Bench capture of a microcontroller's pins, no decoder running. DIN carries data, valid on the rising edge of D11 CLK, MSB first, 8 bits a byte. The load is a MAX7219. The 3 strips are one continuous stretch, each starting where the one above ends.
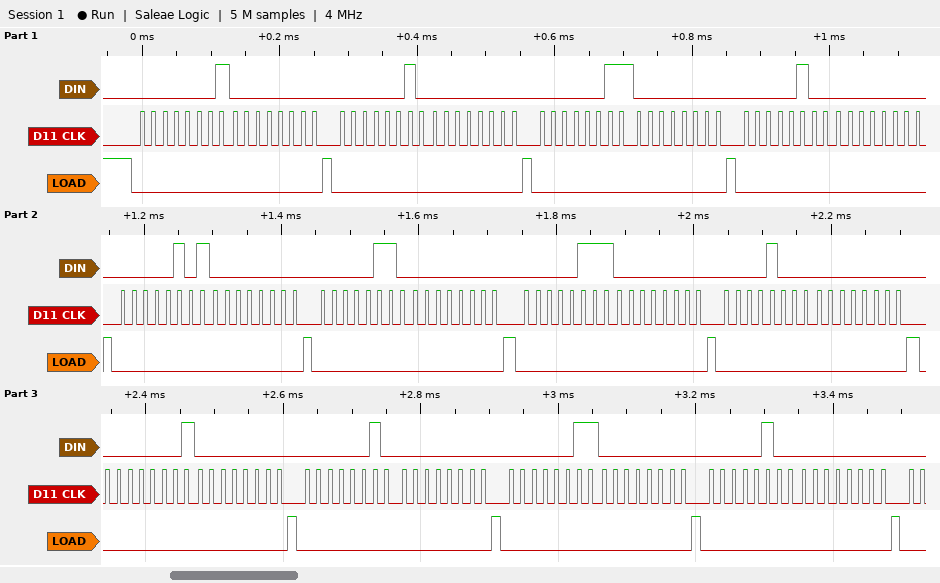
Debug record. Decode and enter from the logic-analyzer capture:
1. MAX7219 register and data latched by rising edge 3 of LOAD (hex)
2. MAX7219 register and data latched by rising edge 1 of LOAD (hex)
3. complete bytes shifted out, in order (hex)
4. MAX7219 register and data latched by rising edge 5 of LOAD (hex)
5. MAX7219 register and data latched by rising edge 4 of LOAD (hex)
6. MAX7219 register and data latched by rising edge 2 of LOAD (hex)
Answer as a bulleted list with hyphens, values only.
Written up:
- register 0x3, data 0x00
- register 0x1, data 0x00
- 01 00 02 00 03 00 04 00 05 00 06 00 07 00 08 00 01 00 02 00 03 00 04 00
- register 0x5, data 0x00
- register 0x4, data 0x00
- register 0x2, data 0x00
